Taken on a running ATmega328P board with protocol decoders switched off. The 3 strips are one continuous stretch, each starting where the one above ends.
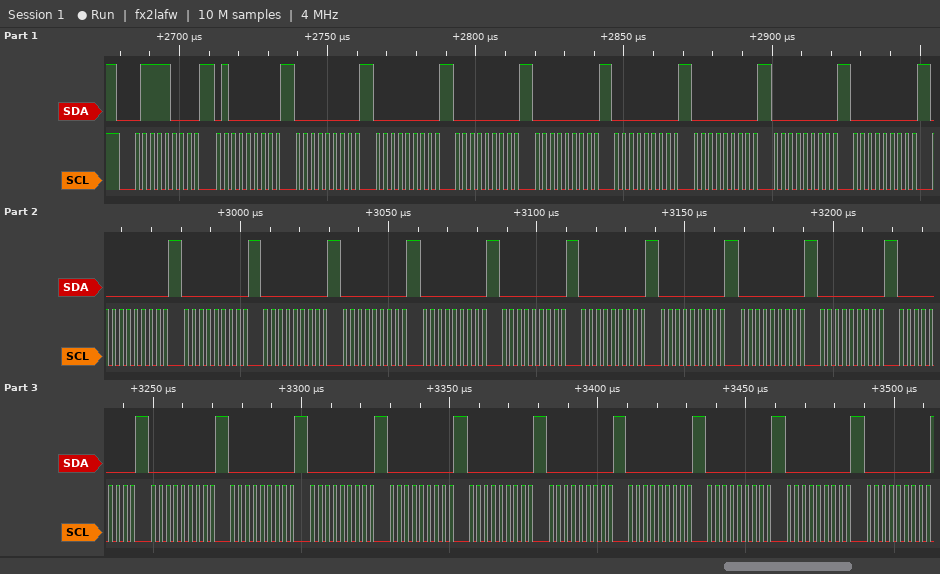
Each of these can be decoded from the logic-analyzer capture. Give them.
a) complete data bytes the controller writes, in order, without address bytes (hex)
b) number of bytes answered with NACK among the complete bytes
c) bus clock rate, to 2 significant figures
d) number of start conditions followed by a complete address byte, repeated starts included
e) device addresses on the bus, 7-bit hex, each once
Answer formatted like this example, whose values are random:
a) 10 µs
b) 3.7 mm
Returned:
a) 40 00 00 00 00 00 00 00 00 00 00 00 00 00 00 00 00 00 00 00 00 00 00 00 00 00 00 00 00 00
b) 0
c) 400 kHz
d) 1
e) 0x3C
